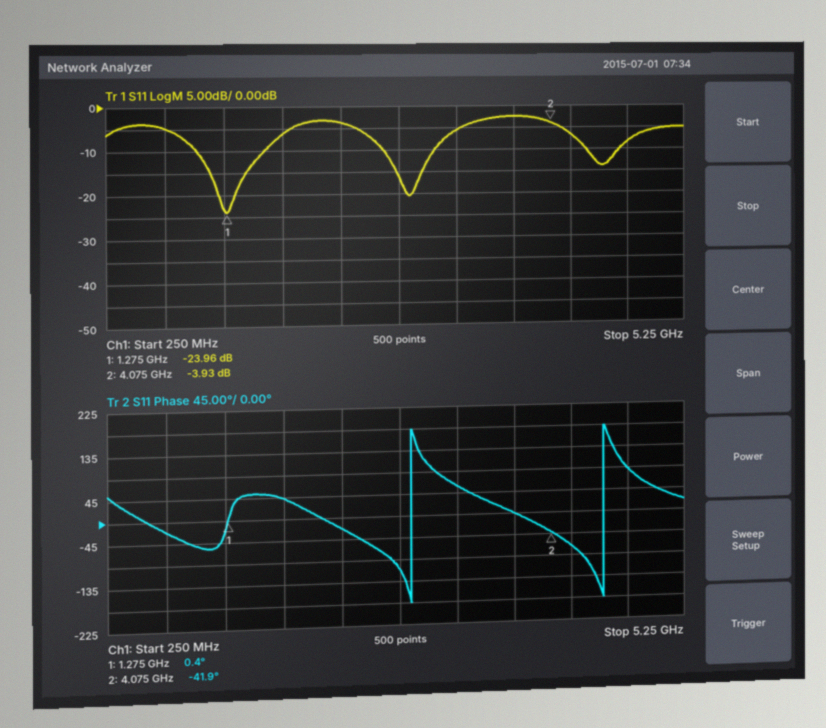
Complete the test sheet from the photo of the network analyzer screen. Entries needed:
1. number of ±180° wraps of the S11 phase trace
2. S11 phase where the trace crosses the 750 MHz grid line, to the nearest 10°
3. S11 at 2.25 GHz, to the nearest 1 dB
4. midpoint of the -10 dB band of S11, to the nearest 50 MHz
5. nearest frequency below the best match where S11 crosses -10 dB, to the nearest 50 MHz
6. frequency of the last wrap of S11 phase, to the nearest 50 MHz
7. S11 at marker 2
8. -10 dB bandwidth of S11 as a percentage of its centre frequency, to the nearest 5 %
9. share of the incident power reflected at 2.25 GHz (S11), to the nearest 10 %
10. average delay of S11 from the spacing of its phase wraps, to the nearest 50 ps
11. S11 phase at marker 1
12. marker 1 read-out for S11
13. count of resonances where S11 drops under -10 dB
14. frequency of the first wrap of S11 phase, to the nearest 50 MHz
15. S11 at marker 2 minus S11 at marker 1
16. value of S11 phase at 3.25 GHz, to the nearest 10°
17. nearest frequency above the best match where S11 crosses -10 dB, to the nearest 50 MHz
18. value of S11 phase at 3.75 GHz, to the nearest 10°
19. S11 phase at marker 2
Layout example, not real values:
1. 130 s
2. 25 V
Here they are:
1. 2
2. -20°
3. -4 dB
4. 1.30 GHz
5. 1.00 GHz
6. 4.55 GHz
7. -3.93 dB
8. 45 %
9. 40 %
10. 600 ps
11. 0.4°
12. -23.96 dB
13. 3
14. 2.85 GHz
15. 20.03 dB
16. 60°
17. 1.60 GHz
18. 0°
19. -41.9°
